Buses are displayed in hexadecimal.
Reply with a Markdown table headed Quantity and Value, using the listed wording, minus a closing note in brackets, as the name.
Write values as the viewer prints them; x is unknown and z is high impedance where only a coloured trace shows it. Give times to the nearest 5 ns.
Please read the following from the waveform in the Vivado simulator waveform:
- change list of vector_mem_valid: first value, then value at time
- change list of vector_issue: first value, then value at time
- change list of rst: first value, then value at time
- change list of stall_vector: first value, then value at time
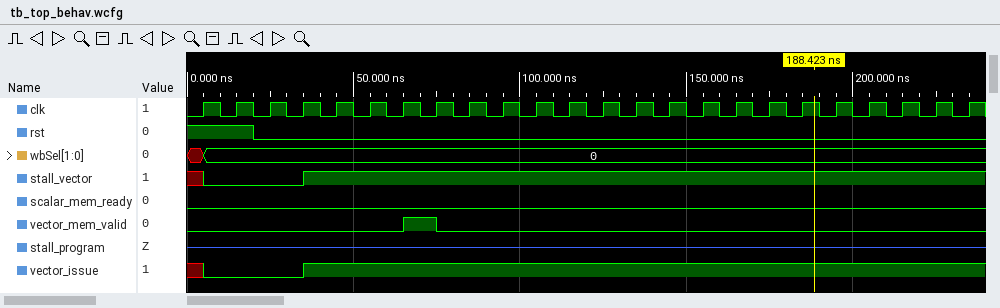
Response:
| Quantity | Value |
|---|---|
| change list of vector_mem_valid: first value, then value at time | 0, 1 at 65 ns, 0 at 75 ns |
| change list of vector_issue: first value, then value at time | x, 0 at 5 ns, 1 at 35 ns |
| change list of rst: first value, then value at time | 1, 0 at 20 ns |
| change list of stall_vector: first value, then value at time | x, 0 at 5 ns, 1 at 35 ns |
